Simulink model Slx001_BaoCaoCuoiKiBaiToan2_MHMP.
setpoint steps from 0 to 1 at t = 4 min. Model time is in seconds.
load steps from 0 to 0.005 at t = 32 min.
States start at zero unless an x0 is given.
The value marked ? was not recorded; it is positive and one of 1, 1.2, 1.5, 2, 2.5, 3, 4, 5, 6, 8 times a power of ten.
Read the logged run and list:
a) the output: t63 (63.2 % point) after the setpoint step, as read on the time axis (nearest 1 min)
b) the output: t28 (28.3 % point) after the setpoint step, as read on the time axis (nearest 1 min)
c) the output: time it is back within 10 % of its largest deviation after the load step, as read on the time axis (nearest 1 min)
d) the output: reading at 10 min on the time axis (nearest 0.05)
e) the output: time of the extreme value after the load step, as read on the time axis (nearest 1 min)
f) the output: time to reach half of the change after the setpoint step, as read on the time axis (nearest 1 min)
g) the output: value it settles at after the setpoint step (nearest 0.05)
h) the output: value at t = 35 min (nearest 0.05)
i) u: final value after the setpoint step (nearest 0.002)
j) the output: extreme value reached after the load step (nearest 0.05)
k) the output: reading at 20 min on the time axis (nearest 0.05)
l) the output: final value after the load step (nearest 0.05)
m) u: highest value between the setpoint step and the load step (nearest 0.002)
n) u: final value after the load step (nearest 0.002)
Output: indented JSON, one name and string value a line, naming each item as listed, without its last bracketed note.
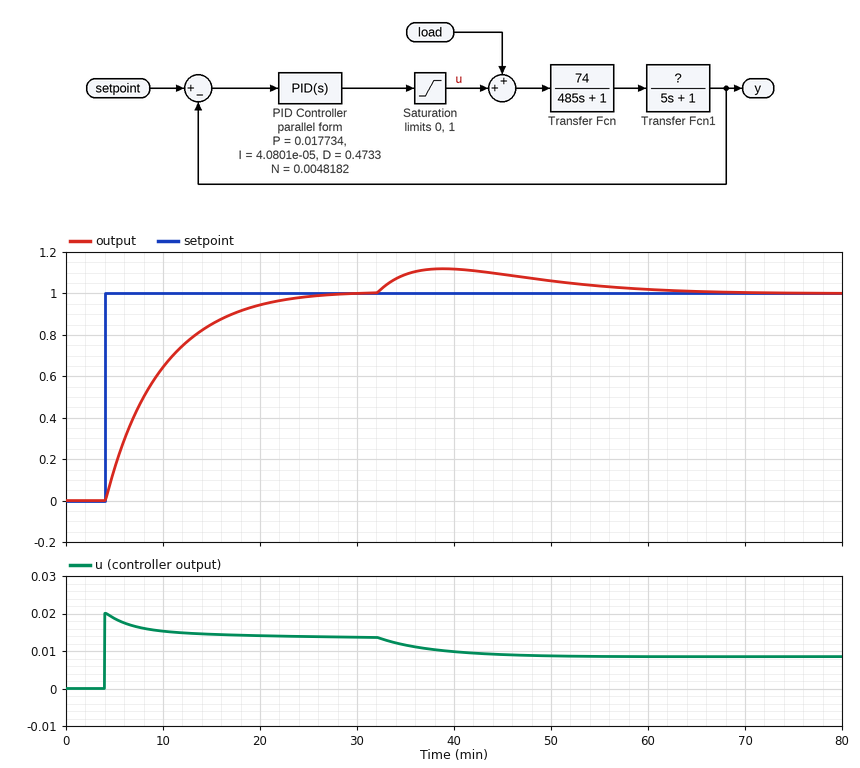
{
  "the output: t63 (63.2 % point) after the setpoint step, as read on the time axis": "10 min",
  "the output: t28 (28.3 % point) after the setpoint step, as read on the time axis": "6 min",
  "the output: time it is back within 10 % of its largest deviation after the load step, as read on the time axis": "64 min",
  "the output: reading at 10 min on the time axis": "0.65",
  "the output: time of the extreme value after the load step, as read on the time axis": "39 min",
  "the output: time to reach half of the change after the setpoint step, as read on the time axis": "8 min",
  "the output: value it settles at after the setpoint step": "1.00",
  "the output: value at t = 35 min": "1.10",
  "u: final value after the setpoint step": "0.014",
  "the output: extreme value reached after the load step": "1.10",
  "the output: reading at 20 min on the time axis": "0.95",
  "the output: final value after the load step": "1.00",
  "u: highest value between the setpoint step and the load step": "0.020",
  "u: final value after the load step": "0.008"
}
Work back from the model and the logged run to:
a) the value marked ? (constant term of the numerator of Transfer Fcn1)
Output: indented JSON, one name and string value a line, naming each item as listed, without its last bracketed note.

{
  "the value marked ?": "1"
}
